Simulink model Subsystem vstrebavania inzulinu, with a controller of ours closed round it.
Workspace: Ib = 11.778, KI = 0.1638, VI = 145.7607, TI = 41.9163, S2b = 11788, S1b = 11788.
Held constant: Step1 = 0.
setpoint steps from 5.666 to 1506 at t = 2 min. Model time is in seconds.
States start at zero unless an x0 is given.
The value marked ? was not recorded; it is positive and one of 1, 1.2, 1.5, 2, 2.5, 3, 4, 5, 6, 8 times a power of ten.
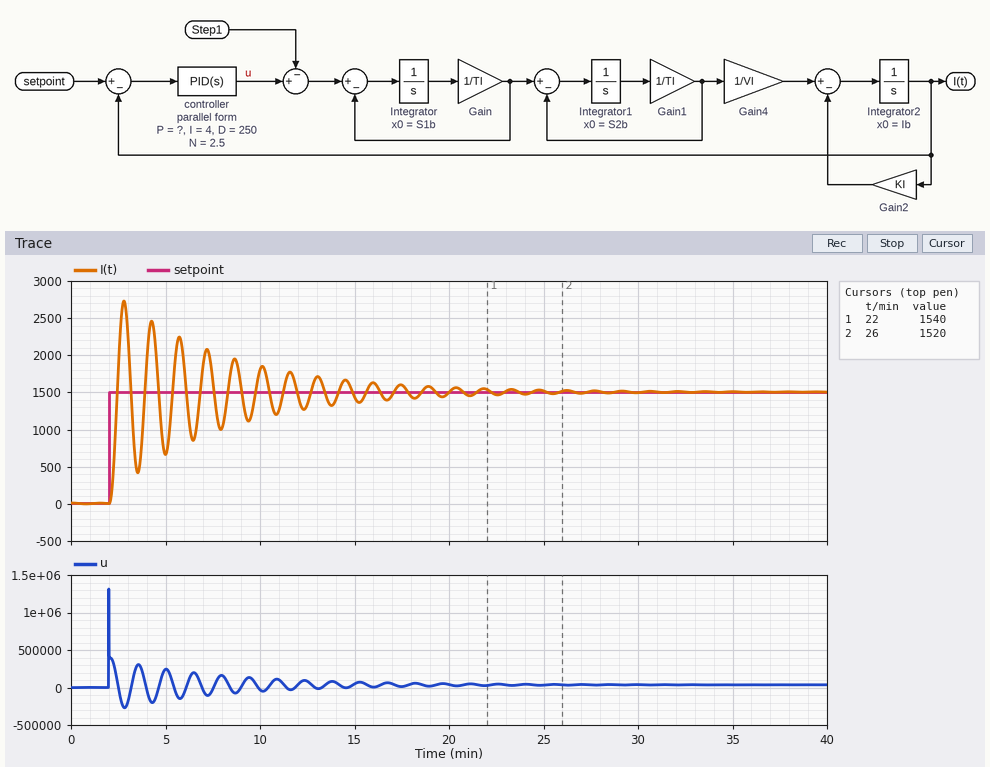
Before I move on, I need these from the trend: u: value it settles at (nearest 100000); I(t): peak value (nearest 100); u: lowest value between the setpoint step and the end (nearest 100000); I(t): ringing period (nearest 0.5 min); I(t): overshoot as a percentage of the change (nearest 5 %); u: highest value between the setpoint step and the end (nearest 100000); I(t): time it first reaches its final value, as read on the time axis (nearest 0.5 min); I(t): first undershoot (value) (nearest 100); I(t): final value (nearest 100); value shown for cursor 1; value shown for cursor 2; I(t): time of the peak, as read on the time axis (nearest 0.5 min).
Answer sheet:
0
2700
-300000
1.5 min
80 %
1300000
2.5 min
400
1500
1540
1520
3.0 min
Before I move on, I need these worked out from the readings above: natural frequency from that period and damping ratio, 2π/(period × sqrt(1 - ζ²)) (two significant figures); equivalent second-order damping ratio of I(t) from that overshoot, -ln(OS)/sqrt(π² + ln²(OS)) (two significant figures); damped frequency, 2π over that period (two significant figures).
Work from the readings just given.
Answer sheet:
4.2 rad/min
0.071
4.2 rad/min
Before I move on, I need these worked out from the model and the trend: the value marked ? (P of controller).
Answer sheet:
250
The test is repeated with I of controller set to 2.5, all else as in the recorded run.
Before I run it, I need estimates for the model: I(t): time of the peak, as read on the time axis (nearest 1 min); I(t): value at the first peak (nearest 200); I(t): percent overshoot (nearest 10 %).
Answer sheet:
3 min
2600
70 %
